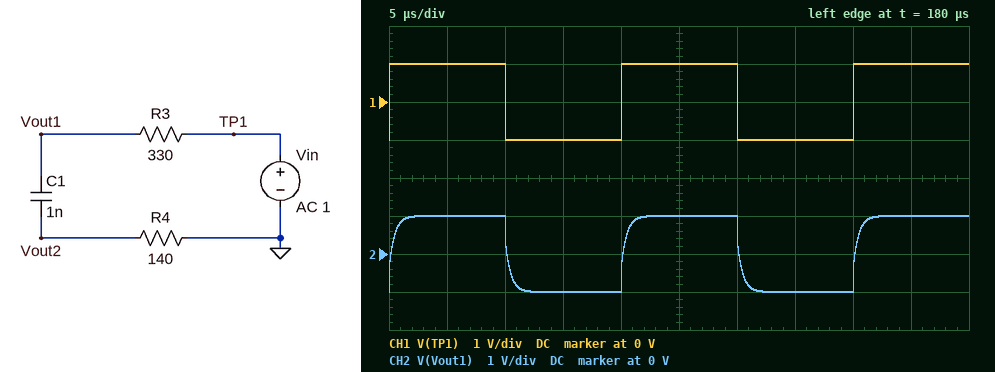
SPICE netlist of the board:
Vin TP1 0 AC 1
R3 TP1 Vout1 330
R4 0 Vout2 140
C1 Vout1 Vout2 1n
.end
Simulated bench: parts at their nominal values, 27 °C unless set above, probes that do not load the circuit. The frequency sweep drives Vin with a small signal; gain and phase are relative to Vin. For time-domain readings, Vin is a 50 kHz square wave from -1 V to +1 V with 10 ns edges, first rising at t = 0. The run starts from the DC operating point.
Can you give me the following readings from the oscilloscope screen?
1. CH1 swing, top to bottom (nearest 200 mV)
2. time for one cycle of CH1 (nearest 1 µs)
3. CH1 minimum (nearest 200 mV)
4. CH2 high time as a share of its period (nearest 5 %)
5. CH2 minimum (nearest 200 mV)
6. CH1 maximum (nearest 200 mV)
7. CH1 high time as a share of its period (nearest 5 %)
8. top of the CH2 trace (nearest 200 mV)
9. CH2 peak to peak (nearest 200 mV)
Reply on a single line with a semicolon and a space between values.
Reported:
2.0 V; 20 µs; -1.0 V; 50 %; -1.0 V; 1.0 V; 50 %; 1.0 V; 2.0 V
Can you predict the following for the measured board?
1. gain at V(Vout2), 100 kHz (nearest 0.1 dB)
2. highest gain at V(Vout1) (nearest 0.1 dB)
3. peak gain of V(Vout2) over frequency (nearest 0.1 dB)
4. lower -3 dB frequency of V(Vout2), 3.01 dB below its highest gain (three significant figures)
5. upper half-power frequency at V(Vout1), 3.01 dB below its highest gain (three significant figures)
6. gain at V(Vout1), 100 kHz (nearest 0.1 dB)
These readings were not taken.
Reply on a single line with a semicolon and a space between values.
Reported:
-21.5 dB; 0 dB; -10.5 dB; 339 kHz; 373 kHz; -0.3 dB
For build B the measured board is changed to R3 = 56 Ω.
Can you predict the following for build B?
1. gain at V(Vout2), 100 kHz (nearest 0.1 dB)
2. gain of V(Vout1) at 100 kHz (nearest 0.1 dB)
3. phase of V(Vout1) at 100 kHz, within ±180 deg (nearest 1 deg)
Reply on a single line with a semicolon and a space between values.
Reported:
-21.2 dB; 0 dB; -2 deg
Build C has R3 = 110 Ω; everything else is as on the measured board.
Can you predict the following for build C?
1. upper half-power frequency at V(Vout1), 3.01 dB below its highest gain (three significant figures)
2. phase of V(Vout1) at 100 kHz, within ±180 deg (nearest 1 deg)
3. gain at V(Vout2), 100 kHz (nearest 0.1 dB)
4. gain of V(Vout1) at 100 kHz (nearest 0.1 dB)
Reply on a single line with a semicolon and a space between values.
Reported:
1.04 MHz; -4 deg; -21.2 dB; -0.1 dB
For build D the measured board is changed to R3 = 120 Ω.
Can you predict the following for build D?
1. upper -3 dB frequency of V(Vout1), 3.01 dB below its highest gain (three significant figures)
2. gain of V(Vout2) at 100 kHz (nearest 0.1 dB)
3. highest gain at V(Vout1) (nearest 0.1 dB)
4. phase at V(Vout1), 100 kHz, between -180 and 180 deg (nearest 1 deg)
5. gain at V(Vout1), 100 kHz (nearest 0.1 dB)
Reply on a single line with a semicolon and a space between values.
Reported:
944 kHz; -21.2 dB; 0 dB; -4 deg; -0.1 dB
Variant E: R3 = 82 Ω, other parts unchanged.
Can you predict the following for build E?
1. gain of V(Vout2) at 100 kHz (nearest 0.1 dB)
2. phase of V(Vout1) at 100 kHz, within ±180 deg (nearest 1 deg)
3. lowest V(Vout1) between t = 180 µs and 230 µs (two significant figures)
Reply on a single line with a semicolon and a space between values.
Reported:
-21.2 dB; -3 deg; -1.0 V
